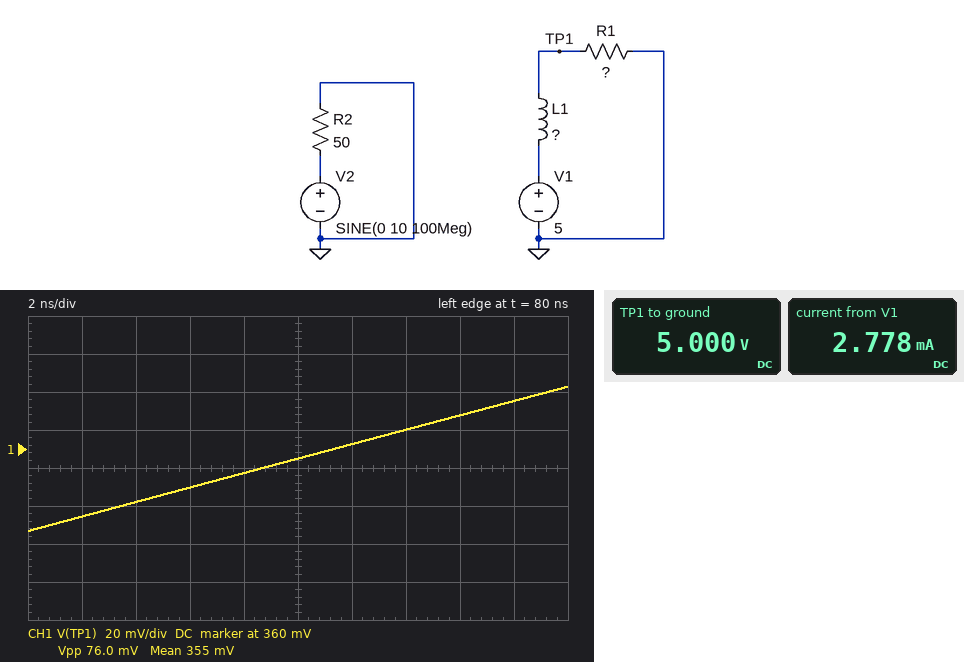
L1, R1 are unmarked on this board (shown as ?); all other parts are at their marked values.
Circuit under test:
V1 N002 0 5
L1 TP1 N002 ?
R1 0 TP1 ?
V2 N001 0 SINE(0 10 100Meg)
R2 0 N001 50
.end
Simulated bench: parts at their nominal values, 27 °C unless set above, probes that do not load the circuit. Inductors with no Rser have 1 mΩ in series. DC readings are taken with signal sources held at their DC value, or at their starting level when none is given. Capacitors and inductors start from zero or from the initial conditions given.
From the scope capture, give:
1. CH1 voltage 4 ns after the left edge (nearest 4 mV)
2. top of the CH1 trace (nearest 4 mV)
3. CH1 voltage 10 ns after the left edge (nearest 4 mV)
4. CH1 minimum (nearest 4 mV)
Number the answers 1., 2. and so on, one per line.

1. 332 mV
2. 392 mV
3. 356 mV
4. 316 mV
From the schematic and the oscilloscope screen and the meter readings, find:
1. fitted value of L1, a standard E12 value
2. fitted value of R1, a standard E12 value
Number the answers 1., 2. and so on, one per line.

1. 2.2 mH
2. 1.8 kΩ
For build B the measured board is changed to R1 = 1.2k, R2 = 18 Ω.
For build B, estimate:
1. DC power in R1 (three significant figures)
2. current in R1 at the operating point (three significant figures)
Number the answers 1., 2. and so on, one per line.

1. 20.8 mW
2. 4.17 mA
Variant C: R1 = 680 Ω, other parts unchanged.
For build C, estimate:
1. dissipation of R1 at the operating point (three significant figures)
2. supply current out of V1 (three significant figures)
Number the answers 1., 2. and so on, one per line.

1. 36.8 mW
2. 7.35 mA
